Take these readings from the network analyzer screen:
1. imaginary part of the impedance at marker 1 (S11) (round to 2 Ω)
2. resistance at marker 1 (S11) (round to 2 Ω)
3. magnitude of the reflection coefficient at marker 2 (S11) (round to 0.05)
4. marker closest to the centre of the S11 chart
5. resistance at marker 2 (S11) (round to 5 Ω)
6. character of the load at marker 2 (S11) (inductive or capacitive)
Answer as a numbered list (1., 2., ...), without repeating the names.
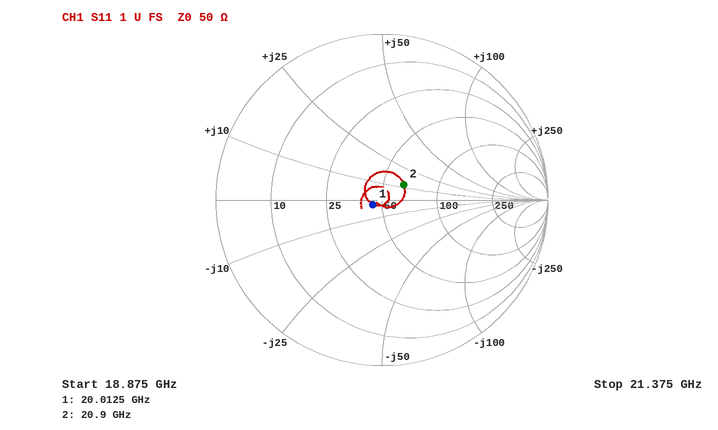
1. -2 Ω
2. 44 Ω
3. 0.15
4. marker 1
5. 65 Ω
6. inductive
